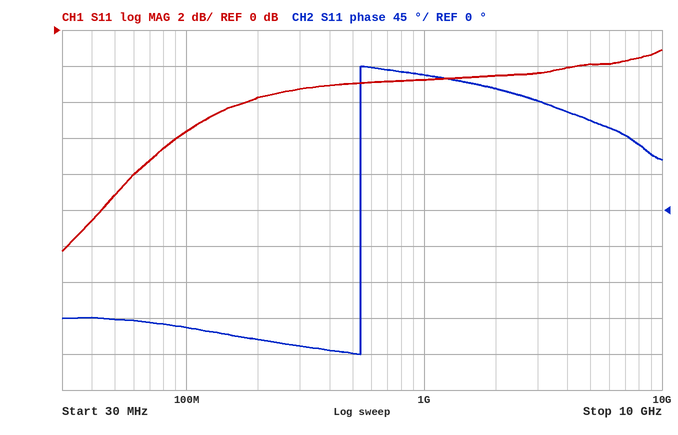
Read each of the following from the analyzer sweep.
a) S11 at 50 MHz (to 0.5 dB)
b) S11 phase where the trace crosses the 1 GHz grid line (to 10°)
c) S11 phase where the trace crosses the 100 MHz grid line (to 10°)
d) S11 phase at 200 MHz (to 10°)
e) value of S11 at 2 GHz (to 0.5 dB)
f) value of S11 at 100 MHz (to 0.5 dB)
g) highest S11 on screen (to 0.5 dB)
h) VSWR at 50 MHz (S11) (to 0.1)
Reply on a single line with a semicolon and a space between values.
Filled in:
-9.0 dB; 170°; -150°; -160°; -2.5 dB; -5.5 dB; -1.0 dB; 2.1
